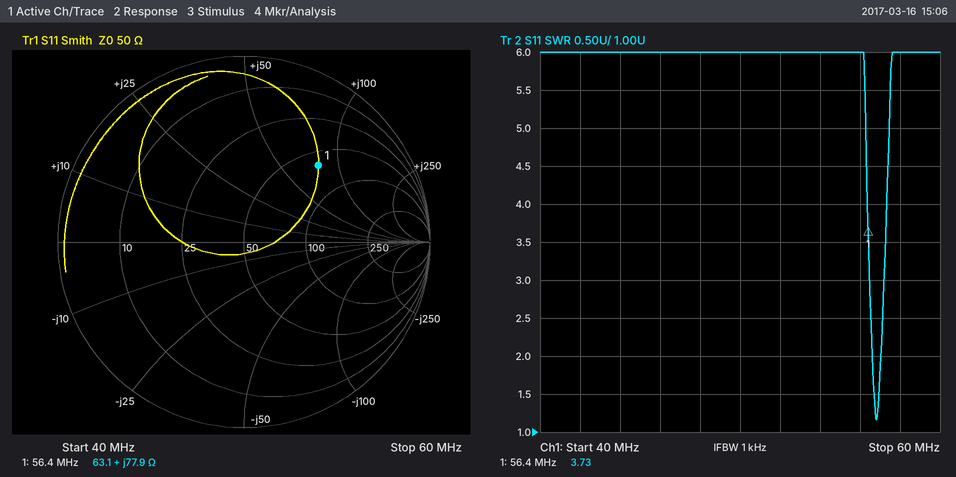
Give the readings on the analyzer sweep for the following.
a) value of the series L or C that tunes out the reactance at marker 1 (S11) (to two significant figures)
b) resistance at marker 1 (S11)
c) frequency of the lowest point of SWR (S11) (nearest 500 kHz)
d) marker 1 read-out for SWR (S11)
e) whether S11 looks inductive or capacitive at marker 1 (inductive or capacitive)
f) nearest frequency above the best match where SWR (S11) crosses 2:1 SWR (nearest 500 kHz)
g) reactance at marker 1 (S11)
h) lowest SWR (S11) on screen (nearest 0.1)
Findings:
36 pF
63.1 Ω
57.0 MHz
3.73
inductive
57.0 MHz
+77.9 Ω
1.2
